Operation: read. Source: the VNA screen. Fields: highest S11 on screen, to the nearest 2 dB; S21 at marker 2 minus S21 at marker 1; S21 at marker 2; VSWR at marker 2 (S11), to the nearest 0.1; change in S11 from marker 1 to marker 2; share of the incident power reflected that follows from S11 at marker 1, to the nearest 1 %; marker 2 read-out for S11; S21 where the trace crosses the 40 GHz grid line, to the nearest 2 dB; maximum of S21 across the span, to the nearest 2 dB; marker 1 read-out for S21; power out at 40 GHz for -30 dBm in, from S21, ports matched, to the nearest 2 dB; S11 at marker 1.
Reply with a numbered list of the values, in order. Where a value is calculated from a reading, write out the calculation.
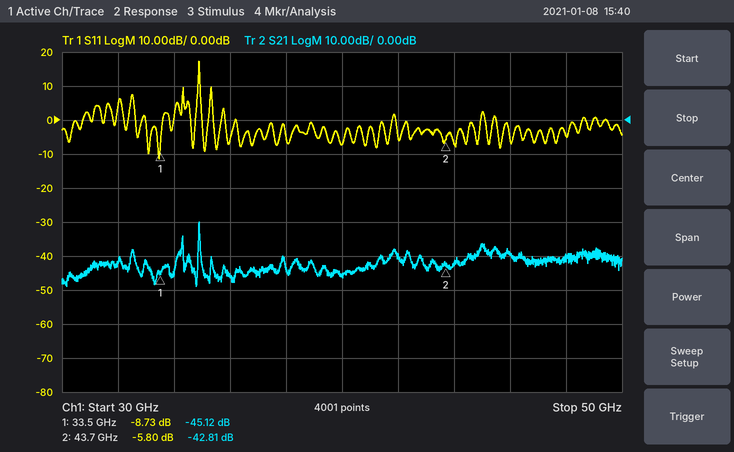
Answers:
1. 18 dB
2. -42.81 − (-45.12) = 2.31 dB
3. -42.81 dB
4. (1 + 0.5129)/(1 − 0.5129) ≈ 3.1
5. -5.8 − (-8.73) = 2.93 dB
6. 10^(-8.73/10) ≈ 13 %
7. -5.80 dB
8. -46 dB
9. -30 dB
10. -45.12 dB
11. -30 dBm + (-46 dB) = -76 dBm
12. -8.73 dB
